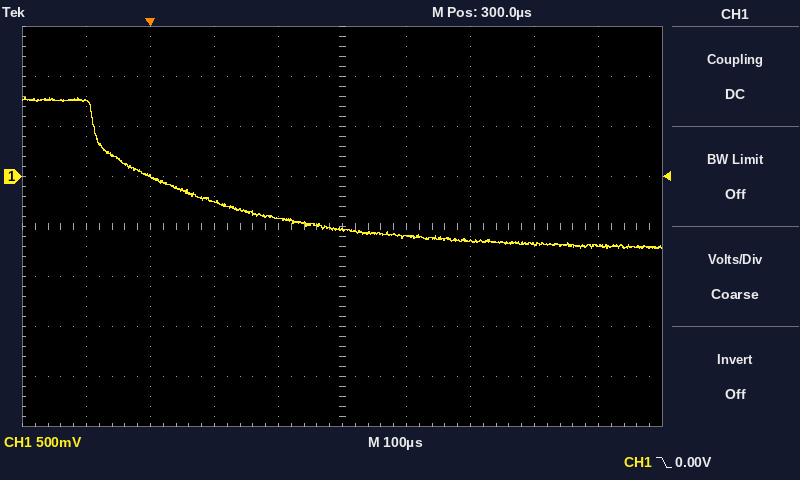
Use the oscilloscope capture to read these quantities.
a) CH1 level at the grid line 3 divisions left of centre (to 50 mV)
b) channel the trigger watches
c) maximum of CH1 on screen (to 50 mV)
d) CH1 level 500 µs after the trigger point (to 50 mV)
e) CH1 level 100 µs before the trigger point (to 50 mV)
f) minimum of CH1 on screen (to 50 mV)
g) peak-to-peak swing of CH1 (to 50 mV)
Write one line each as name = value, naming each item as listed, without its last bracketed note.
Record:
CH1 level at the grid line 3 divisions left of centre = 0 mV
channel the trigger watches = CH1
maximum of CH1 on screen = 800 mV
CH1 level 500 µs after the trigger point = -650 mV
CH1 level 100 µs before the trigger point = 750 mV
minimum of CH1 on screen = -700 mV
peak-to-peak swing of CH1 = 1.50 V
